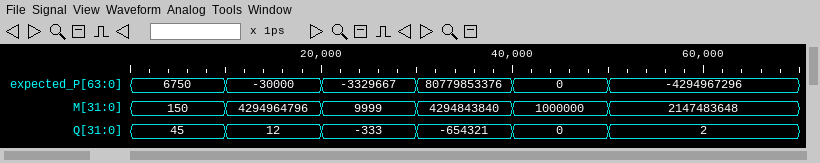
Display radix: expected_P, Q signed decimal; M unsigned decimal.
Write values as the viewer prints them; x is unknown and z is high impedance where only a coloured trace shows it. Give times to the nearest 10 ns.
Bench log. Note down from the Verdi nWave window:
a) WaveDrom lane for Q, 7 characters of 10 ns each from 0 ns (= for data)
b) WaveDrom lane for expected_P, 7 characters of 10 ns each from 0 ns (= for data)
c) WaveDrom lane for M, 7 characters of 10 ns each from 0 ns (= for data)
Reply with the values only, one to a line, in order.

{name: 'Q', wave: '======.', data: '45 12 -333 -654321 0 2'}
{name: 'expected_P', wave: '======.', data: '6750 -30000 -3329667 80779853376 0 -4294967296'}
{name: 'M', wave: '======.', data: '150 4294964796 9999 4294843840 1000000 2147483648'}
